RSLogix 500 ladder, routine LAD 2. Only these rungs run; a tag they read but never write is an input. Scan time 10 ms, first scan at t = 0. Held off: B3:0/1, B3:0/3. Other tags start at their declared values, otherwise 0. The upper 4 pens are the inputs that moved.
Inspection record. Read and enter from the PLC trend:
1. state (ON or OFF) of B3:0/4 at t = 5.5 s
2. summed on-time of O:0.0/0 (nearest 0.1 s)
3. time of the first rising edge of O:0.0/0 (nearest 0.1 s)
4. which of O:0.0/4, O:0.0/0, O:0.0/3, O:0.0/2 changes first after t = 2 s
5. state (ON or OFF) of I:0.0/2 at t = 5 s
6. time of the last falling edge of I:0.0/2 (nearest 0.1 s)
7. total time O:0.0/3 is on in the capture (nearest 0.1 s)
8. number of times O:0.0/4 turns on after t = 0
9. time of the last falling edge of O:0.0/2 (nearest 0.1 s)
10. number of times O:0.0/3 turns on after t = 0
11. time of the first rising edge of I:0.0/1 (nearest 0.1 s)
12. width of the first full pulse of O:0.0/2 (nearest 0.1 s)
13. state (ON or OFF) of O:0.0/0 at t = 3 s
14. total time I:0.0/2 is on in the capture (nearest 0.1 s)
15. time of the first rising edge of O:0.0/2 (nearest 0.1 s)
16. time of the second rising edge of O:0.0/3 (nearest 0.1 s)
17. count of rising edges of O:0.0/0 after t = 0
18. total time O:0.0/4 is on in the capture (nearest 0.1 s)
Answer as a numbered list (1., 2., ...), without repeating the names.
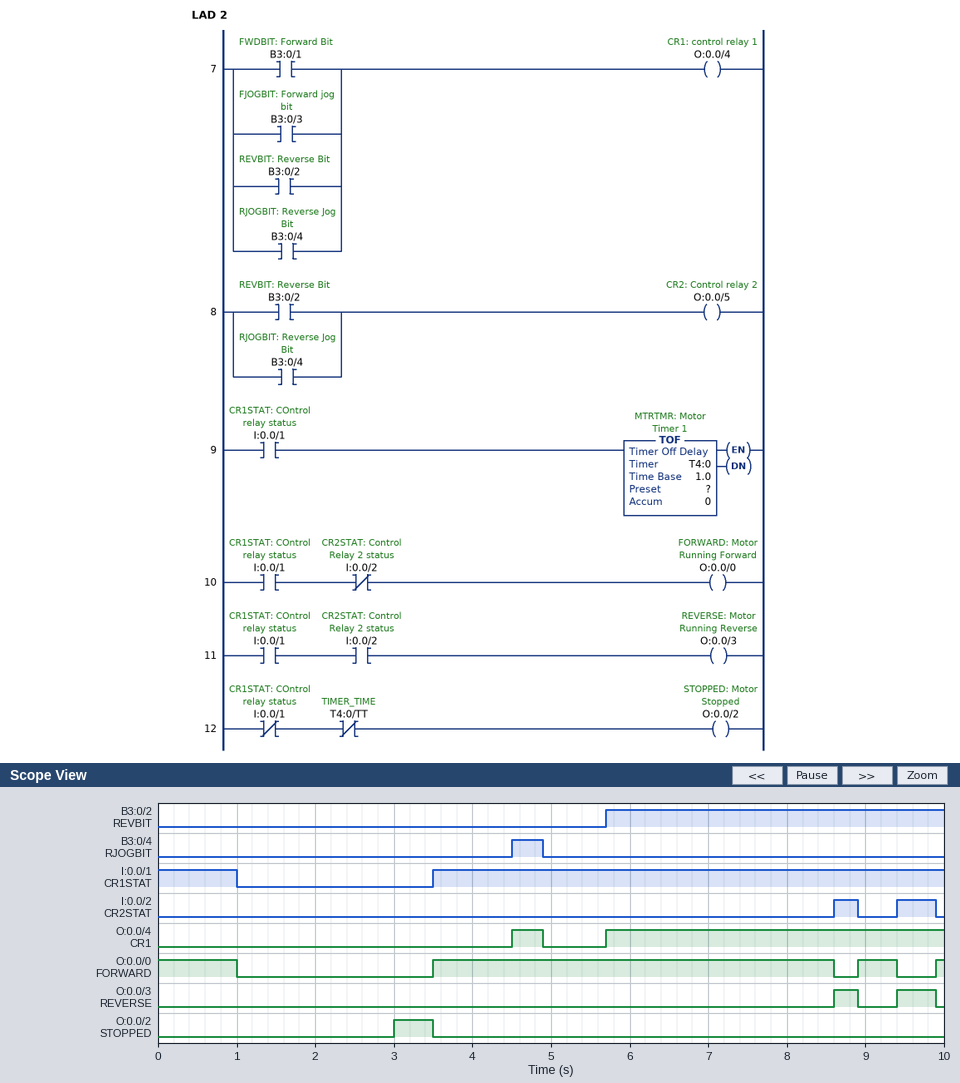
1. OFF
2. 6.7 s
3. 3.5 s
4. O:0.0/2
5. OFF
6. 9.9 s
7. 0.8 s
8. 2
9. 3.5 s
10. 2
11. 3.5 s
12. 0.5 s
13. OFF
14. 0.8 s
15. 3.0 s
16. 9.4 s
17. 3
18. 4.7 s
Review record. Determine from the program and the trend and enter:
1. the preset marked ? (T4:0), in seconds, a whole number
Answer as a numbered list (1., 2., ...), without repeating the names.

1. 2 s
